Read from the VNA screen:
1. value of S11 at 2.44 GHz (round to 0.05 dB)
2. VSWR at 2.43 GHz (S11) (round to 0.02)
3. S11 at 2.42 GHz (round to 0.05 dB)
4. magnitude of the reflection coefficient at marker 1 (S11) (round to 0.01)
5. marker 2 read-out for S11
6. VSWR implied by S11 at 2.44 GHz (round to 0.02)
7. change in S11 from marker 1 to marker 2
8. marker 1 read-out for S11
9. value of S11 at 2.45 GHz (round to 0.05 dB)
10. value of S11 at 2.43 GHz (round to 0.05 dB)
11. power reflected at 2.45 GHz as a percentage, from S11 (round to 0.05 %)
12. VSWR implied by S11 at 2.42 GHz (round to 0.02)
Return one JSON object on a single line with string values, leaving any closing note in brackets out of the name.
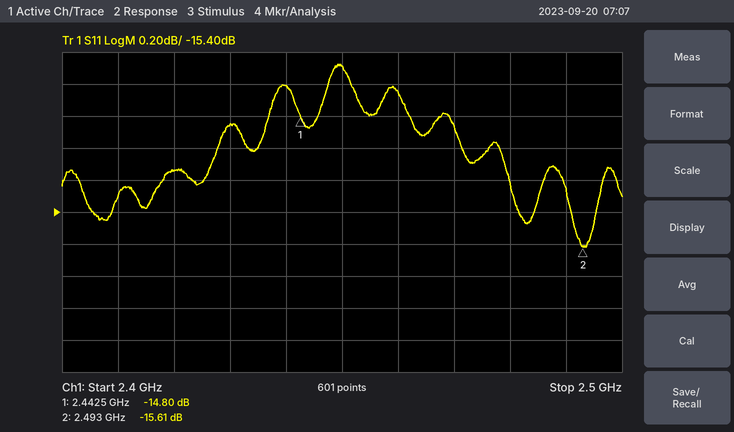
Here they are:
{"value of S11 at 2.44 GHz": "-14.60 dB", "VSWR at 2.43 GHz (S11)": "1.44", "S11 at 2.42 GHz": "-15.15 dB", "magnitude of the reflection coefficient at marker 1 (S11)": "0.18", "marker 2 read-out for S11": "-15.61 dB", "VSWR implied by S11 at 2.44 GHz": "1.46", "change in S11 from marker 1 to marker 2": "-0.81 dB", "marker 1 read-out for S11": "-14.80 dB", "value of S11 at 2.45 GHz": "-14.50 dB", "value of S11 at 2.43 GHz": "-14.85 dB", "power reflected at 2.45 GHz as a percentage, from S11": "3.55 %", "VSWR implied by S11 at 2.42 GHz": "1.42"}
